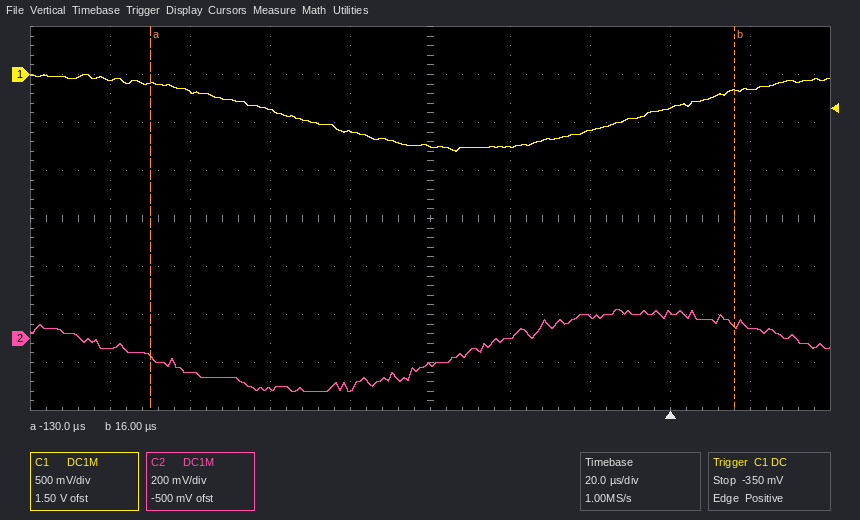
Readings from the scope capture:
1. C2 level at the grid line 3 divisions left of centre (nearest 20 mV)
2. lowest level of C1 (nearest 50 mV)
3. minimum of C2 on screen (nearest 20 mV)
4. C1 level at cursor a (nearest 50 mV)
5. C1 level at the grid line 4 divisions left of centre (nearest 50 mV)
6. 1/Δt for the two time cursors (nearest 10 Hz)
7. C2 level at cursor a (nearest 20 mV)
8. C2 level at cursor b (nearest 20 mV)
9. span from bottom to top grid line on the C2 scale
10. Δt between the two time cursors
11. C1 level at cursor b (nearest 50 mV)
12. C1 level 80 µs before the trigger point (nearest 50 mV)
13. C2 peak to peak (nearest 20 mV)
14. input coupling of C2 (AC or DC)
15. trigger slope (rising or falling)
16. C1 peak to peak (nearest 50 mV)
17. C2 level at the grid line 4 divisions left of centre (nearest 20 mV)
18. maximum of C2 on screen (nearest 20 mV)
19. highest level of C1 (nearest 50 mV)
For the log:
-140 mV
-800 mV
-220 mV
-100 mV
-50 mV
6.85 kHz
-80 mV
60 mV
1.6 V
146 µs
-150 mV
-600 mV
340 mV
DC
rising
800 mV
-40 mV
120 mV
0 mV
